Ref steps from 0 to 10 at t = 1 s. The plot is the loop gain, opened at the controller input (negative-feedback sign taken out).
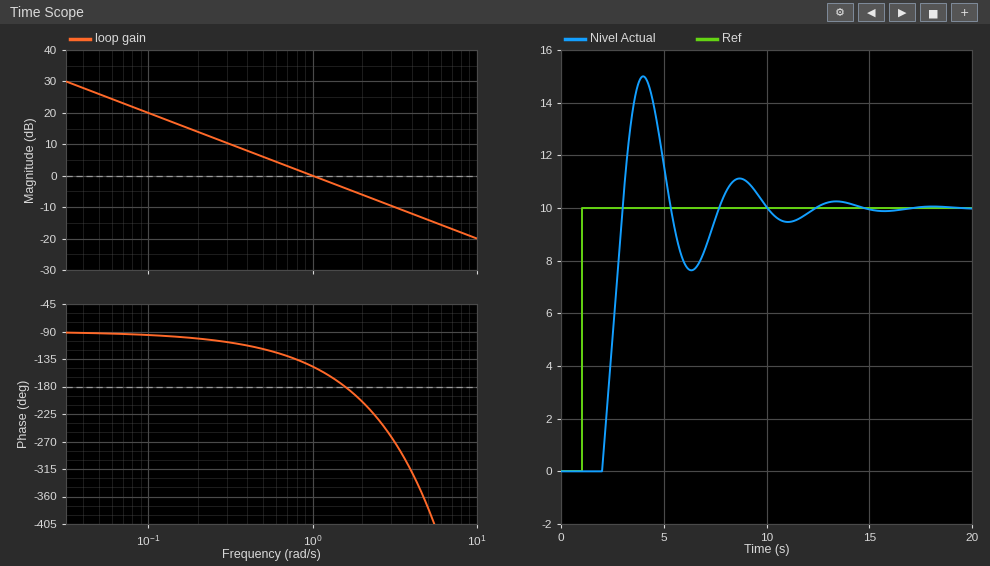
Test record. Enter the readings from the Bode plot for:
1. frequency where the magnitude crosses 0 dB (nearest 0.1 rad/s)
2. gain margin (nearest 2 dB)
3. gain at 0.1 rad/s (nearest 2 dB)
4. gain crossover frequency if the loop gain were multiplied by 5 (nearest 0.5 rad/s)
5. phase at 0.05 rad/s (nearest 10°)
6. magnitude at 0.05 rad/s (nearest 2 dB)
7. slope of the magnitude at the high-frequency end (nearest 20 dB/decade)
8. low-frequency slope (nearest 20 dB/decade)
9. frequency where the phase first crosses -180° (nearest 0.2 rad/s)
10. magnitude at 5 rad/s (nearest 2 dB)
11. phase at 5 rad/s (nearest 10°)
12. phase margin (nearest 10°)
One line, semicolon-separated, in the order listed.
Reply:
1.0 rad/s; 4 dB; 20 dB; 5.0 rad/s; -90°; 26 dB; -20 dB/decade; -20 dB/decade; 1.6 rad/s; -14 dB; -380°; 30°
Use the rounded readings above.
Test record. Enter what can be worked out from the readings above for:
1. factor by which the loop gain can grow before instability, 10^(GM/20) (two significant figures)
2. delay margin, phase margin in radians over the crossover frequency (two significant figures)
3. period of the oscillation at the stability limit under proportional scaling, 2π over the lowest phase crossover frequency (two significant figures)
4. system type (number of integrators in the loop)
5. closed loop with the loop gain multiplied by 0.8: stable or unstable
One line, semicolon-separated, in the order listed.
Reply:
1.6; 0.52 s; 3.9 s; 1; stable
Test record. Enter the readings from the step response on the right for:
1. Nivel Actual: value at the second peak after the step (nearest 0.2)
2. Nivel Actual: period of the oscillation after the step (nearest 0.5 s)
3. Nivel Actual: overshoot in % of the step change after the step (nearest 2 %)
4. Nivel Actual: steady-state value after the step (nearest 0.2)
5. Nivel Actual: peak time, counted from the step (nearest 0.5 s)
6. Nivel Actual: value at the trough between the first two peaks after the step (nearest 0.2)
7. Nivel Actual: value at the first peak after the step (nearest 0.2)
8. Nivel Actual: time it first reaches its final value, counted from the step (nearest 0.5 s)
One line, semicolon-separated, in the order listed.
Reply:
11.2; 4.5 s; 50 %; 10.0; 3.0 s; 7.6; 15.0; 2.0 s
